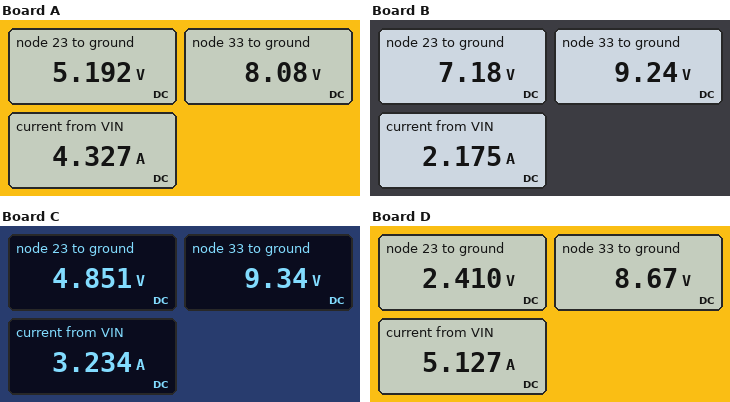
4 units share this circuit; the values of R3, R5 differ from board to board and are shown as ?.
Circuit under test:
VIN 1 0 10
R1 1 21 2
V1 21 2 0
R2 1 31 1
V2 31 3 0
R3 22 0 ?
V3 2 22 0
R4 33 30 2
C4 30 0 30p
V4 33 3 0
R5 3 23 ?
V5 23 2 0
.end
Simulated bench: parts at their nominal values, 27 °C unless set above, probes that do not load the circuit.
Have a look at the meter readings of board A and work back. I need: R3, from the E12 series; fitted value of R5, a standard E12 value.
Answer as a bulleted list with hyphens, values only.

- 1.2 Ω
- 1.5 Ω
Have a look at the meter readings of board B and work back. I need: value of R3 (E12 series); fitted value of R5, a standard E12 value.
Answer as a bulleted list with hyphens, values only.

- 3.3 Ω
- 2.7 Ω
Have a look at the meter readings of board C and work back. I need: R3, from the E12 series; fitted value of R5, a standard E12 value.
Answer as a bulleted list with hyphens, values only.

- 1.5 Ω
- 6.8 Ω
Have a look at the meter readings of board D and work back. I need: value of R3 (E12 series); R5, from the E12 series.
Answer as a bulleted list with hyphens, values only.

- 0.47 Ω
- 4.7 Ω
